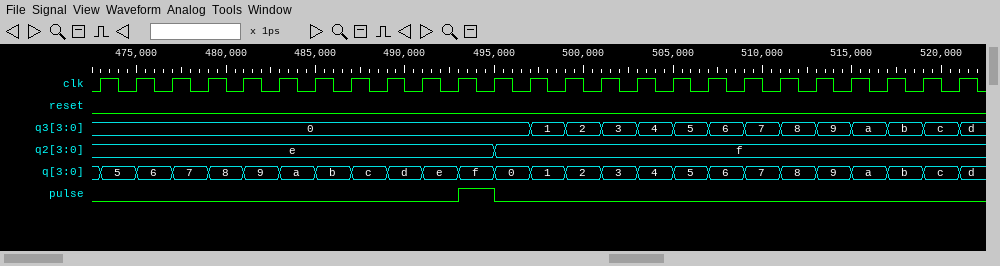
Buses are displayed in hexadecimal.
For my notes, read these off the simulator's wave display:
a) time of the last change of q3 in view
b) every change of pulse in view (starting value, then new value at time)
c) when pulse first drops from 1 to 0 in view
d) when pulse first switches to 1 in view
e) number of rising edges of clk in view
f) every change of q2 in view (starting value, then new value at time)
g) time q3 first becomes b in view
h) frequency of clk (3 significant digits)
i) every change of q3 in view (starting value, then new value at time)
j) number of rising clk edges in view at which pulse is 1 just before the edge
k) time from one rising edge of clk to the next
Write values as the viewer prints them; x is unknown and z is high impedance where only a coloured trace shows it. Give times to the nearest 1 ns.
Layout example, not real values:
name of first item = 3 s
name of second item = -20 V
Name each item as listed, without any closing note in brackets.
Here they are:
time of the last change of q3 in view = 521 ns
every change of pulse in view = 0, 1 at 493 ns, 0 at 495 ns
when pulse first drops from 1 to 0 in view = 495 ns
when pulse first switches to 1 in view = 493 ns
number of rising edges of clk in view = 25
every change of q2 in view = e, f at 495 ns
time q3 first becomes b in view = 517 ns
frequency of clk = 500 MHz
every change of q3 in view = 0, 1 at 497 ns, 2 at 499 ns, 3 at 501 ns, 4 at 503 ns, 5 at 505 ns, 6 at 507 ns, 7 at 509 ns, 8 at 511 ns, 9 at 513 ns, a at 515 ns, b at 517 ns, c at 519 ns, d at 521 ns
number of rising clk edges in view at which pulse is 1 just before the edge = 1
time from one rising edge of clk to the next = 2 ns
